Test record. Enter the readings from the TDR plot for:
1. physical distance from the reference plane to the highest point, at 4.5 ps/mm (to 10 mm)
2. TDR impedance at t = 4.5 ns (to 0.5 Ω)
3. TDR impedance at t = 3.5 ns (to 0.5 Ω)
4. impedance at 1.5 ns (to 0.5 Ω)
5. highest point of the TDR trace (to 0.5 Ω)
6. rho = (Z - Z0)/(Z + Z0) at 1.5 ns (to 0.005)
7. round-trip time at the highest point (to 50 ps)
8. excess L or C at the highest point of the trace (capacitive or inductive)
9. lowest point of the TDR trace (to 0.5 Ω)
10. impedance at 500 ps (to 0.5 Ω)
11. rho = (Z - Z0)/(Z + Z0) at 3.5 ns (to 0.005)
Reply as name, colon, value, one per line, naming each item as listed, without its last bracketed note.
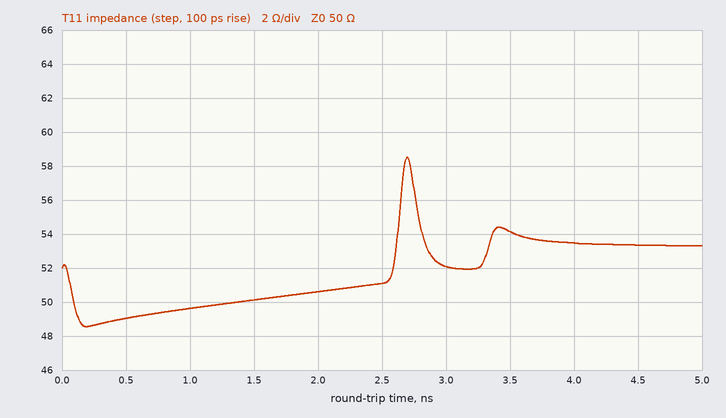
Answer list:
physical distance from the reference plane to the highest point, at 4.5 ps/mm: 300 mm
TDR impedance at t = 4.5 ns: 53.5 Ω
TDR impedance at t = 3.5 ns: 54.0 Ω
impedance at 1.5 ns: 50.0 Ω
highest point of the TDR trace: 58.5 Ω
rho = (Z - Z0)/(Z + Z0) at 1.5 ns: 0.000
round-trip time at the highest point: 2.70 ns
excess L or C at the highest point of the trace: inductive
lowest point of the TDR trace: 48.5 Ω
impedance at 500 ps: 49.0 Ω
rho = (Z - Z0)/(Z + Z0) at 3.5 ns: +0.040
